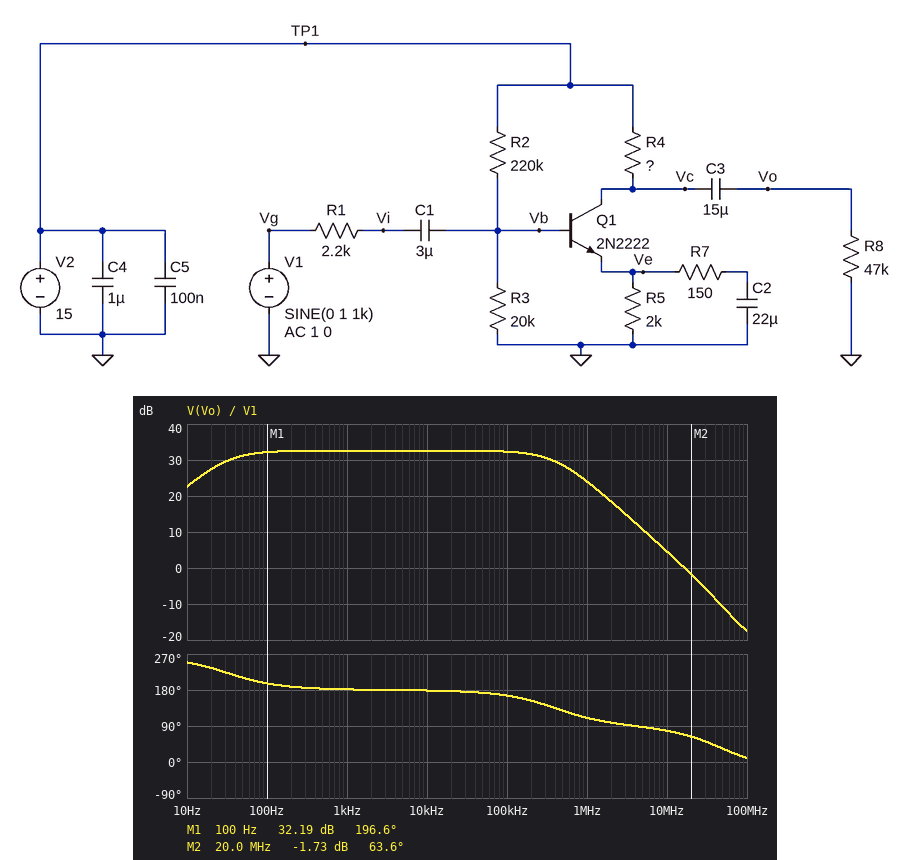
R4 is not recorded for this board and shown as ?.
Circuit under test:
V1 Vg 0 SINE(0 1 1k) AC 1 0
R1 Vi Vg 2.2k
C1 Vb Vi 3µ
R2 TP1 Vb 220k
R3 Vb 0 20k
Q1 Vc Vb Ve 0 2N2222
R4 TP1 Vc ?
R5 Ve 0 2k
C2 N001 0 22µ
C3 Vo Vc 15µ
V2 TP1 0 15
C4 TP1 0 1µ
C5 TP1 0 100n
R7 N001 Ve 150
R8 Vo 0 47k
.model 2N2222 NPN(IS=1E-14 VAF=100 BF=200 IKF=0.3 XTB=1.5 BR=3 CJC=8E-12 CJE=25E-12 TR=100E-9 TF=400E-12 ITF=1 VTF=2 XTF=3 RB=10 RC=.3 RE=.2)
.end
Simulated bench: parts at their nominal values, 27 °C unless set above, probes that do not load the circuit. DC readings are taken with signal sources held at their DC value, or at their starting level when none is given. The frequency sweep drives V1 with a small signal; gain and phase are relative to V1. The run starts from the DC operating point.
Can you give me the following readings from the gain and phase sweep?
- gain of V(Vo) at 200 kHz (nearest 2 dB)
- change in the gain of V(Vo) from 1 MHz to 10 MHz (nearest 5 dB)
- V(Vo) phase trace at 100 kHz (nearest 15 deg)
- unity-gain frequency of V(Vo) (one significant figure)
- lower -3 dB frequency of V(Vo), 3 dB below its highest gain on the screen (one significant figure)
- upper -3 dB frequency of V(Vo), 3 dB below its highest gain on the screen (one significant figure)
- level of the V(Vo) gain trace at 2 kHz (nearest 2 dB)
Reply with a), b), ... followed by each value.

a) 32 dB
b) -20 dB
c) 165 deg
d) 20 MHz
e) 30 Hz
f) 400 kHz
g) 32 dB
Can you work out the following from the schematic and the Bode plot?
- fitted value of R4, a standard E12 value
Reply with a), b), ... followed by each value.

a) 15 kΩ
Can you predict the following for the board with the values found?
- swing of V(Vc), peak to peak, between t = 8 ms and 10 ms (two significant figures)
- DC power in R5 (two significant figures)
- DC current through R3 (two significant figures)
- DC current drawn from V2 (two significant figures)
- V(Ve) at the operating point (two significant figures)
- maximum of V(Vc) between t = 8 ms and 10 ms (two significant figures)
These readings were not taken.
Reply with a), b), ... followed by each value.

a) 13 V
b) 180 µW
c) 61 µA
d) 360 µA
e) 600 mV
f) 14 V
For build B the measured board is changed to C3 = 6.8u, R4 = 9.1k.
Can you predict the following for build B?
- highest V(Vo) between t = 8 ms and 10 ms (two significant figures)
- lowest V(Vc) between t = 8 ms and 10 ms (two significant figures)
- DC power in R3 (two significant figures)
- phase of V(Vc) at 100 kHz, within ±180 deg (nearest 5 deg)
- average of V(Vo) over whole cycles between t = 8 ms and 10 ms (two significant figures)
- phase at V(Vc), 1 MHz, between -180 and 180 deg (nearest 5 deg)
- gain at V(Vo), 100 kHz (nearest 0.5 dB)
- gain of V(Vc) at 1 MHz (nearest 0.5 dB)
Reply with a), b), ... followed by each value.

a) 2.4 V
b) 1.0 V
c) 75 µW
d) 170 deg
e) -2.5 V
f) 120 deg
g) 29.0 dB
h) 23.5 dB
